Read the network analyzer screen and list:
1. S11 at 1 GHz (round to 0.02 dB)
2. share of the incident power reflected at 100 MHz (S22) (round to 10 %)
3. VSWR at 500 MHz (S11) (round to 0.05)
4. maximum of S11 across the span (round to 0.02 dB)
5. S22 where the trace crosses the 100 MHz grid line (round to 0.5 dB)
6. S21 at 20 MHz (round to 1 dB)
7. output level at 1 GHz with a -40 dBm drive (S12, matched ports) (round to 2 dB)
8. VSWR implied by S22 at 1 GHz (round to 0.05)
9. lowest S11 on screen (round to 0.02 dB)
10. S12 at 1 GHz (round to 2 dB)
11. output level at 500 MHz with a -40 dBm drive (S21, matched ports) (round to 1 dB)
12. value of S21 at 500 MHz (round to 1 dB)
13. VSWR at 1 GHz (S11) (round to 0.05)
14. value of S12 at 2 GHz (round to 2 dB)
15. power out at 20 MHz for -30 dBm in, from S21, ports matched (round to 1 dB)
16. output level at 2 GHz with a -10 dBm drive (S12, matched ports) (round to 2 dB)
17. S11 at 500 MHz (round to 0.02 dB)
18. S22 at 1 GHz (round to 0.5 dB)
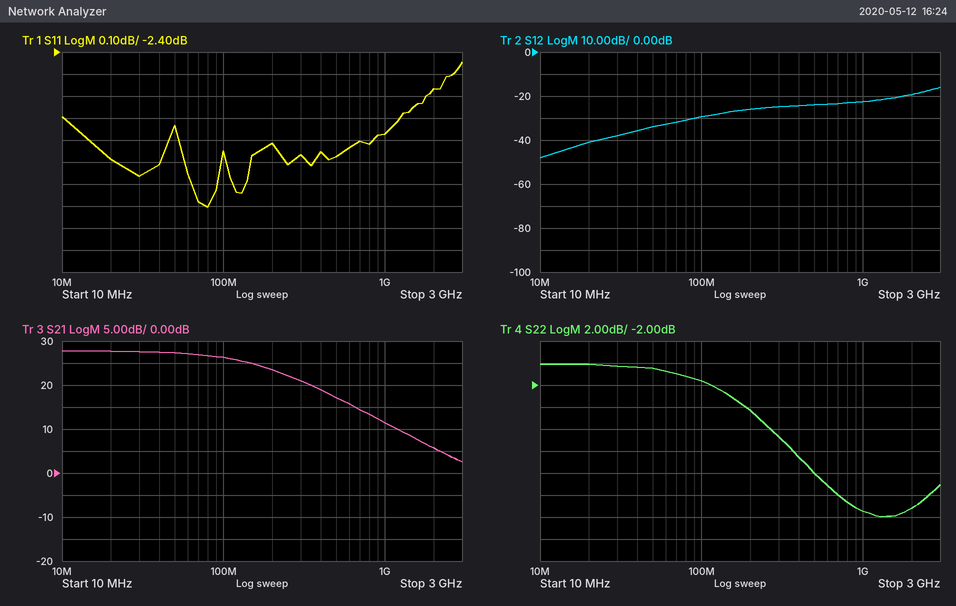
-2.78 dB
70 %
6.10
-2.44 dB
-1.5 dB
28 dB
-62 dBm
1.55
-3.10 dB
-22 dB
-23 dBm
17 dB
6.30
-20 dB
-2 dBm
-30 dBm
-2.88 dB
-13.5 dB
